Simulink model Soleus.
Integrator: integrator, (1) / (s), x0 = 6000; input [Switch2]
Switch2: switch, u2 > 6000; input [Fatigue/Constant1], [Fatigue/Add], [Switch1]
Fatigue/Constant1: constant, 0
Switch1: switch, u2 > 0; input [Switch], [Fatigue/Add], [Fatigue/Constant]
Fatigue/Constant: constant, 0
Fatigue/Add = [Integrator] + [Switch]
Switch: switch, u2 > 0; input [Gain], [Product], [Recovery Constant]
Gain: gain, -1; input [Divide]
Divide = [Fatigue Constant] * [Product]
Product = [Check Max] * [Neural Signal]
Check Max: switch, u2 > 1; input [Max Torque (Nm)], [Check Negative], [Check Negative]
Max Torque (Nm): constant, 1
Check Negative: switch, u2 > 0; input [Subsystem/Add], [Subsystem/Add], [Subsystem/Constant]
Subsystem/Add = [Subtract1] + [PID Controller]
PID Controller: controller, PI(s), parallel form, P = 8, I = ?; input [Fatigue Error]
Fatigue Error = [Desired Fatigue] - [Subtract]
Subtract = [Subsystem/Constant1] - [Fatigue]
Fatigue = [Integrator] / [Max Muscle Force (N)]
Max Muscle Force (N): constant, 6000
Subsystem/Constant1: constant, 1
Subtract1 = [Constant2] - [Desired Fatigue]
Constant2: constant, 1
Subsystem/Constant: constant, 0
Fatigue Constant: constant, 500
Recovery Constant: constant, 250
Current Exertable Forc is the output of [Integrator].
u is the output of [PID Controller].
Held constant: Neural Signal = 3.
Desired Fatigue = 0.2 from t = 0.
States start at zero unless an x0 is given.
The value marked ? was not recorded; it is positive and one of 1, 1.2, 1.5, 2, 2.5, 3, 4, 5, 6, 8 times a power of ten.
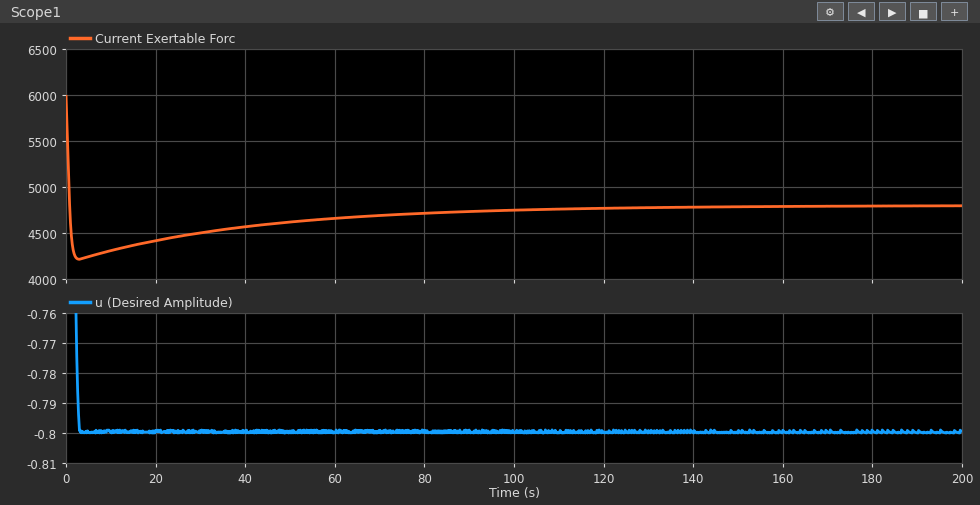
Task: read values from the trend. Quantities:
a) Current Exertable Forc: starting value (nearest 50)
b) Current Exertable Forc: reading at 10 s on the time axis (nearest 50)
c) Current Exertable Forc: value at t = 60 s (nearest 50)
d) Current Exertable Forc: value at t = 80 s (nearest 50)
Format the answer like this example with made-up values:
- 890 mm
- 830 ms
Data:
- 6000
- 4300
- 4650
- 4700
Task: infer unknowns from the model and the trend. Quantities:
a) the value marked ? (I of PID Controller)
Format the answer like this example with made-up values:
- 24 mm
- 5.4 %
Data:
- 0.2
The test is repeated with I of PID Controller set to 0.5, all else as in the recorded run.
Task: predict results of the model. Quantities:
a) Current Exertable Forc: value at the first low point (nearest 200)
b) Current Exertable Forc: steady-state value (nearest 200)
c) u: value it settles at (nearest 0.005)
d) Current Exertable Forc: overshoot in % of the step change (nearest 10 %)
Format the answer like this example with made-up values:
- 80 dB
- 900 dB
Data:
- 4200
- 4800
- -0.800
- 50 %
